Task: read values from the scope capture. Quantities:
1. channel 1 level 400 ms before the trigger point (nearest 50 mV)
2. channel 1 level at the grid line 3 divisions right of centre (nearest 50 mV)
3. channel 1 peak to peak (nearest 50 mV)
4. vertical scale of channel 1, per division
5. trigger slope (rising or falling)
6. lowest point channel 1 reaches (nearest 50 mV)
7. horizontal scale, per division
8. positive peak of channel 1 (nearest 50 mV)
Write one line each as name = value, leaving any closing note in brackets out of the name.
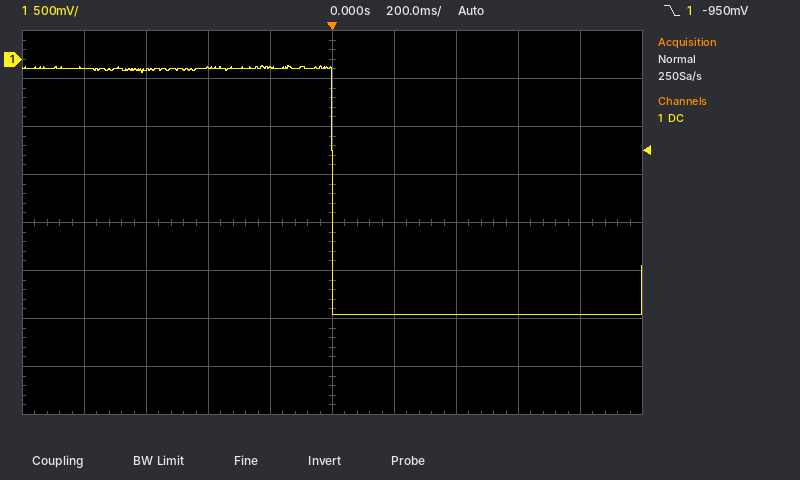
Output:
channel 1 level 400 ms before the trigger point = -100 mV
channel 1 level at the grid line 3 divisions right of centre = -2.65 V
channel 1 peak to peak = 2.60 V
vertical scale of channel 1, per division = 500 mV
trigger slope = falling
lowest point channel 1 reaches = -2.65 V
horizontal scale, per division = 200 ms
positive peak of channel 1 = -50 mV
